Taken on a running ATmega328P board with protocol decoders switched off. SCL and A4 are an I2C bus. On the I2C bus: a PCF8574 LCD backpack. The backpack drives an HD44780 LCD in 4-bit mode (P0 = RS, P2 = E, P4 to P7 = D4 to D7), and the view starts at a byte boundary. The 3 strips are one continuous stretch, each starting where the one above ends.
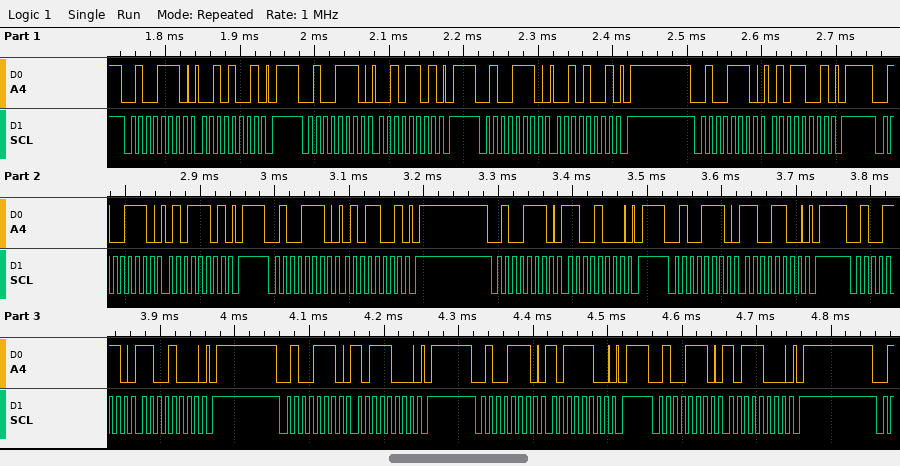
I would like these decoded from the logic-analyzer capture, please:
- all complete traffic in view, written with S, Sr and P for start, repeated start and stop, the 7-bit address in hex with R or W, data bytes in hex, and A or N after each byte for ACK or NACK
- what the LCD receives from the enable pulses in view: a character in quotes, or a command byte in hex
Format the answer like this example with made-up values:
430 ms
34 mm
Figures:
S 27W A 29 A P S 27W A 2D A P S 27W A 29 A P S 27W A 59 A P S 27W A 5D A P S 27W A 59 A P S 27W A C8 A P S 27W A CC A P S 27W A C8 A P S 27W A B8 A P S 27W A BC A P S 27W A B8 A P
'%' 0xCB
